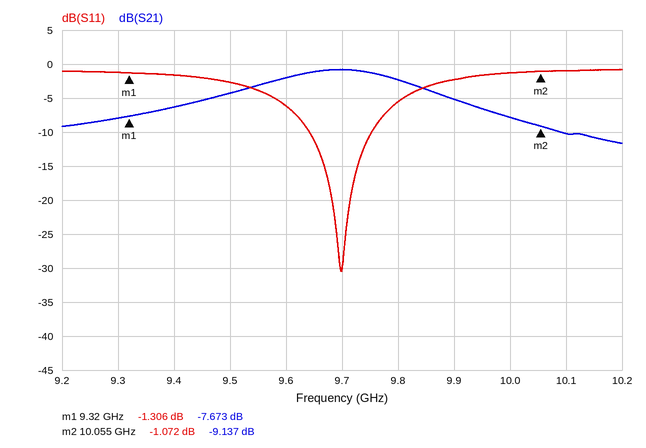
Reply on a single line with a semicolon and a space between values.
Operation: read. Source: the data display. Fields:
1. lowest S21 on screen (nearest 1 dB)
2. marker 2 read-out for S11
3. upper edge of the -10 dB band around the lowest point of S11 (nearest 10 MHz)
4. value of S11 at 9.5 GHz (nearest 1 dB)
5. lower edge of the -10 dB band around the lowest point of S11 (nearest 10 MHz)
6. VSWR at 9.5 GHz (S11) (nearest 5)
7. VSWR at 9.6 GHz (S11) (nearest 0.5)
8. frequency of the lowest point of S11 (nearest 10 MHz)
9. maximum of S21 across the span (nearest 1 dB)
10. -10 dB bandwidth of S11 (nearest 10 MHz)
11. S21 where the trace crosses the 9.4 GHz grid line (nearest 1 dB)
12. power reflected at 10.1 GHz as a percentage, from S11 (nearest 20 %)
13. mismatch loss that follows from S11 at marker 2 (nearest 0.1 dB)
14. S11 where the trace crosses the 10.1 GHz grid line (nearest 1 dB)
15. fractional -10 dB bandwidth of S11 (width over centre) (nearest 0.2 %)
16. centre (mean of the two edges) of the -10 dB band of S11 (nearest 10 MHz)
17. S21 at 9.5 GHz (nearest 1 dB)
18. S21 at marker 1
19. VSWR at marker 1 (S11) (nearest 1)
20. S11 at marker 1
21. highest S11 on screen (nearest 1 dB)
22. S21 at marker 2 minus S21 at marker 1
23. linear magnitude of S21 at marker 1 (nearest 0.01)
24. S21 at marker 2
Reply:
-12 dB; -1.072 dB; 9.75 GHz; -3 dB; 9.64 GHz; 5; 3.0; 9.70 GHz; -1 dB; 110 MHz; -6 dB; 80 %; 6.6 dB; -1 dB; 1.2 %; 9.70 GHz; -4 dB; -7.673 dB; 13; -1.306 dB; -1 dB; -1.464 dB; 0.41; -9.137 dB
